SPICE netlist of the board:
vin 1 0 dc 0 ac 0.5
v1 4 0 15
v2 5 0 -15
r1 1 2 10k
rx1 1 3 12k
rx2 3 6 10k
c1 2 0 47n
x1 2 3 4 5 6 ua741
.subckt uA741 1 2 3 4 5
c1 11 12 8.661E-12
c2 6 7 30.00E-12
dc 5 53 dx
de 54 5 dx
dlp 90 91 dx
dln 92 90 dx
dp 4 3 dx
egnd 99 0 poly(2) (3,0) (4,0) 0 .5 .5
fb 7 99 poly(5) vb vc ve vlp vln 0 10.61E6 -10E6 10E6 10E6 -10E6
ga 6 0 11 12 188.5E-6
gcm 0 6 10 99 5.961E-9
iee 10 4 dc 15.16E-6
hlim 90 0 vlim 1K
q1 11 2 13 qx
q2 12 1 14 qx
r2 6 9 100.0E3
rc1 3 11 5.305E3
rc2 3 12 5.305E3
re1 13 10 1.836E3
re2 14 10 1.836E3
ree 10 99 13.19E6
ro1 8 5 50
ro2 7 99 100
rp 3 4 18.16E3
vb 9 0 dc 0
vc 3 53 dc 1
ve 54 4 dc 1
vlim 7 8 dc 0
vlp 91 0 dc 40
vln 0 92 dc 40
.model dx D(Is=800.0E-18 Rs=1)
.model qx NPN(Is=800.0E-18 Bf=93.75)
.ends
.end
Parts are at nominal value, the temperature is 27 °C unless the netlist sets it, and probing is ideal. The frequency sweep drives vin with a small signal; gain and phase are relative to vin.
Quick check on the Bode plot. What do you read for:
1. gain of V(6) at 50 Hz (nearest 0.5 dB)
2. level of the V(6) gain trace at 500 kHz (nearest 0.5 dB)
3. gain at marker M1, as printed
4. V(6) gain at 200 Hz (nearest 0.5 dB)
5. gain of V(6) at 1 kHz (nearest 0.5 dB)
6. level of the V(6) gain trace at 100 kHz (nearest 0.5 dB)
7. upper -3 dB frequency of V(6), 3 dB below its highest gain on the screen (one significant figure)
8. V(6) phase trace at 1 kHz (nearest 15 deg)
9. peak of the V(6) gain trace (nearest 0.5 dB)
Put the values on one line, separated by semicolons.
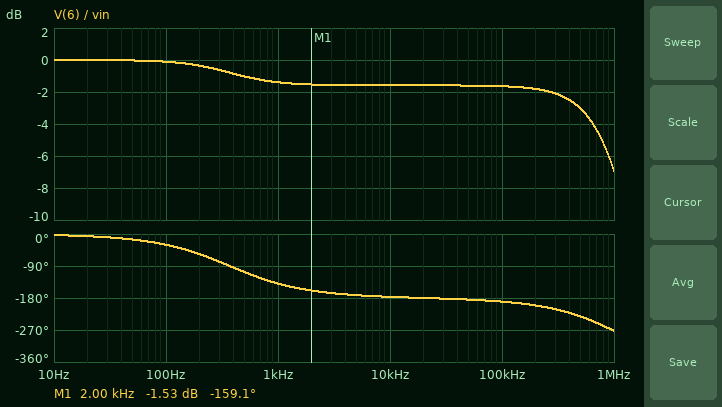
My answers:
0 dB; -3.0 dB; -1.53 dB; -0.5 dB; -1.5 dB; -1.5 dB; 500 kHz; -135 deg; 0 dB
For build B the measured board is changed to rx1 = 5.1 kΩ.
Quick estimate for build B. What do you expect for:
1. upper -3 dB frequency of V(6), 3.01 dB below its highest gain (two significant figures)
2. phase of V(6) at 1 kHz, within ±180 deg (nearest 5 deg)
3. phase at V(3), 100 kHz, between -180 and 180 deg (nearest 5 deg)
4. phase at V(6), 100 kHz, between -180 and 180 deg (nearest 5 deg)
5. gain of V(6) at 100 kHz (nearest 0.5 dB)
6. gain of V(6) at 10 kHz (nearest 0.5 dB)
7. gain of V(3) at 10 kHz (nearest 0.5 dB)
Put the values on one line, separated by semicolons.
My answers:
410 kHz; -150 deg; 75 deg; 165 deg; 5.5 dB; 6.0 dB; -37.0 dB
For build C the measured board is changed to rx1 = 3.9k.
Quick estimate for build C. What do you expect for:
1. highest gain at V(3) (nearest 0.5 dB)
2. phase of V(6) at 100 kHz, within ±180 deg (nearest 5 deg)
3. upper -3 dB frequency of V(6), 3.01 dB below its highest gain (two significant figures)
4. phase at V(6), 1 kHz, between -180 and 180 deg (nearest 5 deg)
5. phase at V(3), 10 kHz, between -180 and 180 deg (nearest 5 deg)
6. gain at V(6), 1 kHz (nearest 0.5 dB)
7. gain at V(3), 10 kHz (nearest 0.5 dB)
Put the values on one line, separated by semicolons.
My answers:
0 dB; 160 deg; 330 kHz; -155 deg; -85 deg; 8.0 dB; -42.0 dB
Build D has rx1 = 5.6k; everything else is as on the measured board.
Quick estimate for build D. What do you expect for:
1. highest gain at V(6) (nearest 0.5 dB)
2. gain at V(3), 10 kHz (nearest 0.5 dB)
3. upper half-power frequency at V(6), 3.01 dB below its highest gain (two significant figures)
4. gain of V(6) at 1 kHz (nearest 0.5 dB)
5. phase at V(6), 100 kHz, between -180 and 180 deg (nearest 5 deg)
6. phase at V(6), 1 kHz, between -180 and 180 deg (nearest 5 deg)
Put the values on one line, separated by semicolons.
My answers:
5.0 dB; -36.0 dB; 440 kHz; 4.5 dB; 165 deg; -150 deg
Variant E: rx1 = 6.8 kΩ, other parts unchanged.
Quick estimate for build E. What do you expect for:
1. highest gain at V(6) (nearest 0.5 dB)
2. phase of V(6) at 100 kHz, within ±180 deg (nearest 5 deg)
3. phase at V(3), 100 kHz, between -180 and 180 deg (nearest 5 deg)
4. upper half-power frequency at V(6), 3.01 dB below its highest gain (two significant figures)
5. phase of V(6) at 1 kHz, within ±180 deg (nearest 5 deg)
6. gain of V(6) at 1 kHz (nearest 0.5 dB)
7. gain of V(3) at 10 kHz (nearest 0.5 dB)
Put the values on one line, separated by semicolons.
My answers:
3.5 dB; 165 deg; 80 deg; 510 kHz; -150 deg; 3.0 dB; -34.5 dB
